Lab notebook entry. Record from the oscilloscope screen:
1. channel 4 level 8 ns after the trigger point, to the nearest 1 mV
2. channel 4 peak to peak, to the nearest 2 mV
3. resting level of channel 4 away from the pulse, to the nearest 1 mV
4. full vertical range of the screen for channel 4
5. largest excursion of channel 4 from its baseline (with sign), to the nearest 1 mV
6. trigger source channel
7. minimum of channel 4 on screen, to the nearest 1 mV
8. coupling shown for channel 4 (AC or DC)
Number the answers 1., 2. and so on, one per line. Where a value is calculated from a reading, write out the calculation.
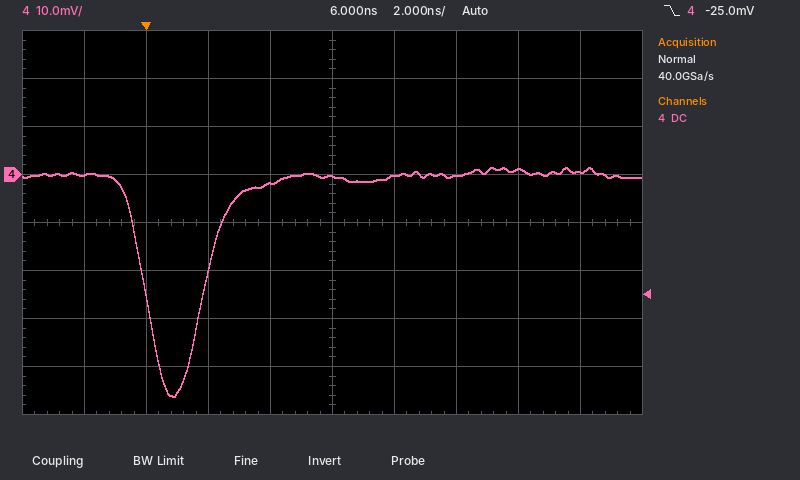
1. 0 mV
2. 48 mV
3. 0 mV
4. 80 mV
5. -46 mV − (0 mV) = -46 mV
6. channel 4
7. -46 mV
8. DC
